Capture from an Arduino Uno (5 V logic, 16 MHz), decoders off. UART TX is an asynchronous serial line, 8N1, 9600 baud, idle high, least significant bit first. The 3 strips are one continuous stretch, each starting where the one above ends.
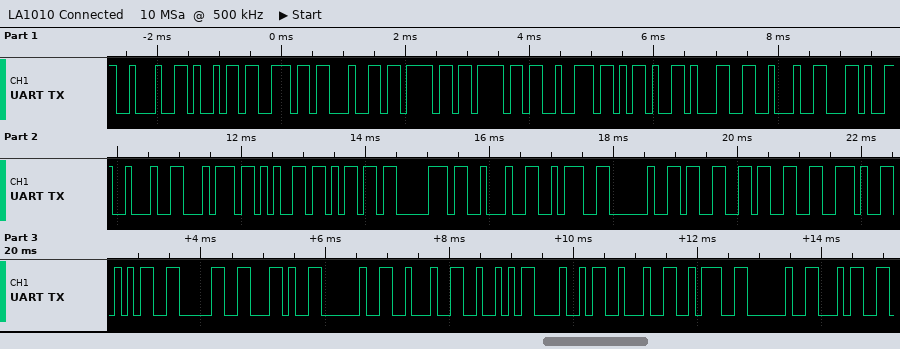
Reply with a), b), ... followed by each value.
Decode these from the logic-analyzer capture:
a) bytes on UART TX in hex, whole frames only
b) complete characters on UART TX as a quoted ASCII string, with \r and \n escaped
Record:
a) 22 69 6E 64 6F 6F 72 2D 31 22 2C 22 74 65 6D 70 22 3A 20 33 33 2E 35 30 2C 20 22 52 48 22 3A 20 34
b) "\"indoor-1\",\"temp\": 33.50, \"RH\": 4"
